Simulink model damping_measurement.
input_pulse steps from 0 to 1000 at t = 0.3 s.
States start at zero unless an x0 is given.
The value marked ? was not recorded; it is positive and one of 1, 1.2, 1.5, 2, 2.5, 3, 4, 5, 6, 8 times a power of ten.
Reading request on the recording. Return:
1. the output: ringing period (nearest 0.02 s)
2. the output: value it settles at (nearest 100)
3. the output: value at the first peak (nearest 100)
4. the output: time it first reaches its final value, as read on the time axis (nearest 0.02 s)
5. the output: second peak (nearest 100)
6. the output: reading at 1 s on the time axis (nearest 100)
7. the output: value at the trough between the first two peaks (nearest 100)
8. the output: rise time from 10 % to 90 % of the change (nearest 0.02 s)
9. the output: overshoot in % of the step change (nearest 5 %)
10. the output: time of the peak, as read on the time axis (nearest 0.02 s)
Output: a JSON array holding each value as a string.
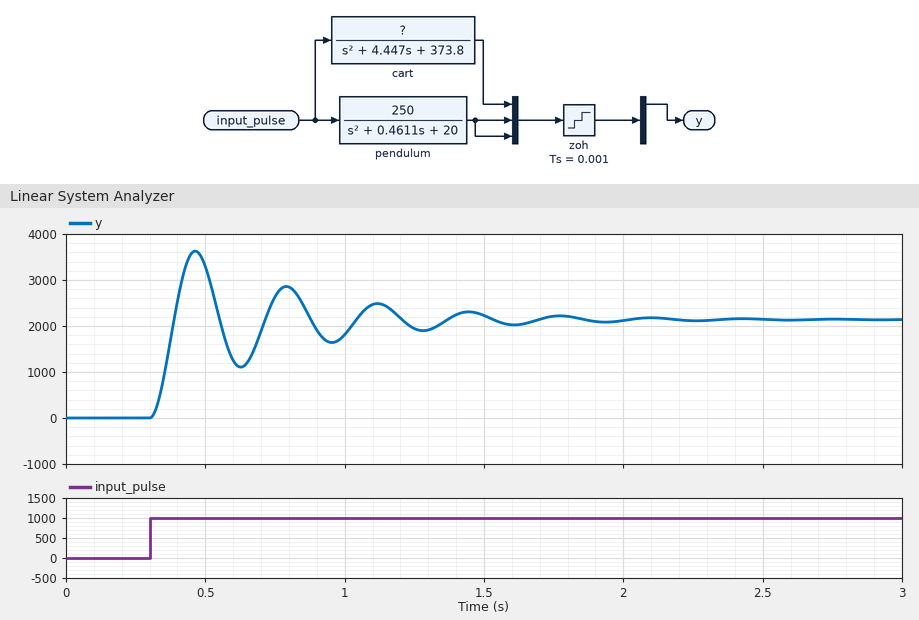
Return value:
["0.32 s", "2100", "3600", "0.38 s", "2900", "1800", "1100", "0.06 s", "70 %", "0.46 s"]
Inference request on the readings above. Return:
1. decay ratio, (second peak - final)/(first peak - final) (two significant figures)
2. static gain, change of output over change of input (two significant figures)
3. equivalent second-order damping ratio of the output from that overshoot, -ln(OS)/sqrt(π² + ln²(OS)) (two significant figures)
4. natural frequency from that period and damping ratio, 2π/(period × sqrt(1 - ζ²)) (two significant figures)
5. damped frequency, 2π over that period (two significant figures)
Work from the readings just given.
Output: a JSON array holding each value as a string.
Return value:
["0.53", "2.1", "0.11", "20 rad/s", "20 rad/s"]
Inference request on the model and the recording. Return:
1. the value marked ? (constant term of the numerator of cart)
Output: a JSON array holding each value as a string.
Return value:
["800"]
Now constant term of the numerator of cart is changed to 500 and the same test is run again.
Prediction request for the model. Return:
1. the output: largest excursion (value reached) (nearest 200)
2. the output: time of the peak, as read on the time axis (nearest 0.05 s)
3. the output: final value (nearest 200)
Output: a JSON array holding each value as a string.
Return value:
["2200", "0.45 s", "1400"]
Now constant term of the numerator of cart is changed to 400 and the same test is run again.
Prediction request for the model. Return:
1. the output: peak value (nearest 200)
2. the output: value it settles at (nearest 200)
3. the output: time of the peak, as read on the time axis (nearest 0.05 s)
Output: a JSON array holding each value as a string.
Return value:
["1800", "1000", "0.45 s"]
